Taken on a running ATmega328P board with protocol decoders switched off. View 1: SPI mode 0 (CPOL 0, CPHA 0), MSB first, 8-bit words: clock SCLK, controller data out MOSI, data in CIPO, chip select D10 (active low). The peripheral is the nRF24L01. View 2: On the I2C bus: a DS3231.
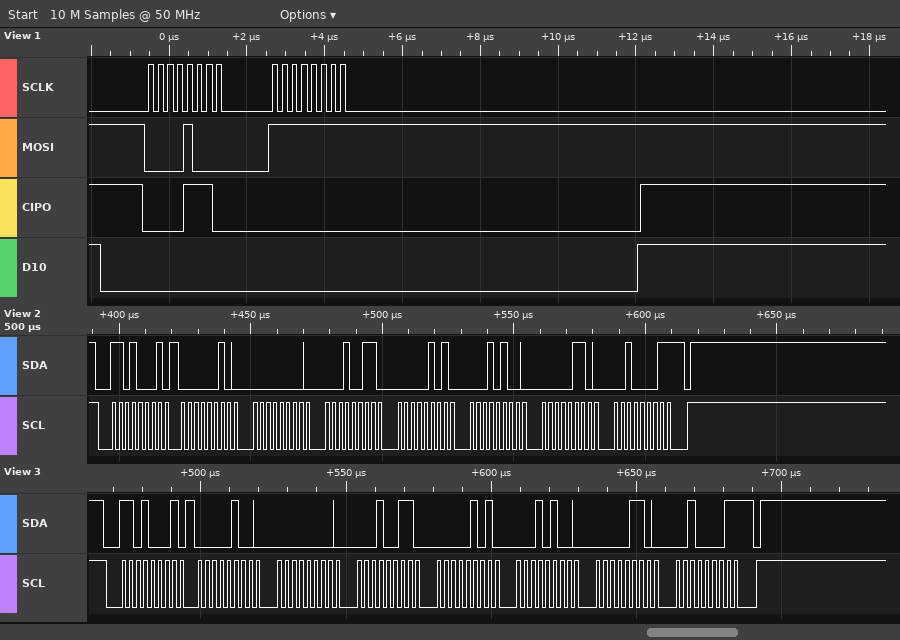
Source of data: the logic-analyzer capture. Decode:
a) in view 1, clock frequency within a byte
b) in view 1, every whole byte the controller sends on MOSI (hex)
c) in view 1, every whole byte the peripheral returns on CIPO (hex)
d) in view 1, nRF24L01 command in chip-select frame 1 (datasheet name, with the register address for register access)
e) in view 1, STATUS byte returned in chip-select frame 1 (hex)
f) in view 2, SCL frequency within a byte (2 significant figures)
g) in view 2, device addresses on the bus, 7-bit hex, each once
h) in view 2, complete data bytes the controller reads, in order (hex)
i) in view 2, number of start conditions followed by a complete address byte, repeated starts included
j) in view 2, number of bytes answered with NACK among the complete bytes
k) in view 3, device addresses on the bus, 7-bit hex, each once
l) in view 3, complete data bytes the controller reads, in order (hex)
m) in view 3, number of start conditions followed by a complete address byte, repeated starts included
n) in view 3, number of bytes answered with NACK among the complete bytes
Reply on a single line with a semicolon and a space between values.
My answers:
4 MHz; 08 FF; 0E 00; R_REGISTER 0x08; 0x0E; 400 kHz; 0x68; 02 00 13 05 14 06 21; 1; 1; 0x68; 04 00 13 05 14 06 21; 1; 1
